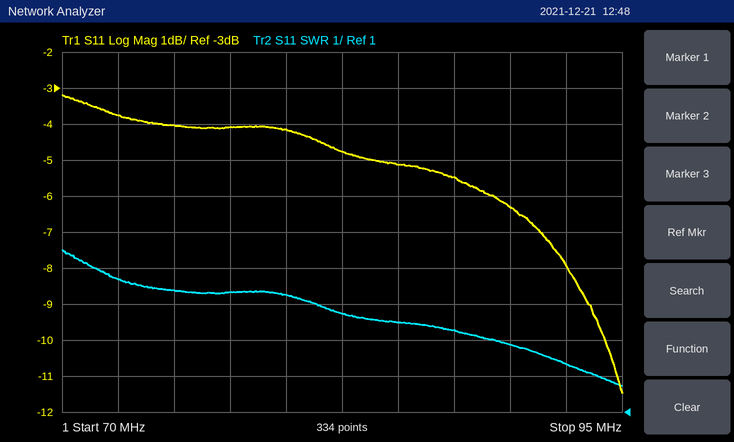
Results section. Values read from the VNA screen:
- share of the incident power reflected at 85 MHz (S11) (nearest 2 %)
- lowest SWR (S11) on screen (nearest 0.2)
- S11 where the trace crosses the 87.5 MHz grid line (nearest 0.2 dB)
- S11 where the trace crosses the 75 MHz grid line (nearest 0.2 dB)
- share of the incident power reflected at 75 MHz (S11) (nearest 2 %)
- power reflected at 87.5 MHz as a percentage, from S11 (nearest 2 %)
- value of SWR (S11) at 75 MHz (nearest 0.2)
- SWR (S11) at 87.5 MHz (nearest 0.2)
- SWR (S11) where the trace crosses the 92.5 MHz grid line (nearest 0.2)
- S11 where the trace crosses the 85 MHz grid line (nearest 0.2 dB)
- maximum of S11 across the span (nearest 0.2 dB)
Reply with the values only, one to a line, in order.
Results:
30 %
1.8
-5.4 dB
-4.0 dB
40 %
28 %
4.4
3.2
2.4
-5.2 dB
-3.2 dB
